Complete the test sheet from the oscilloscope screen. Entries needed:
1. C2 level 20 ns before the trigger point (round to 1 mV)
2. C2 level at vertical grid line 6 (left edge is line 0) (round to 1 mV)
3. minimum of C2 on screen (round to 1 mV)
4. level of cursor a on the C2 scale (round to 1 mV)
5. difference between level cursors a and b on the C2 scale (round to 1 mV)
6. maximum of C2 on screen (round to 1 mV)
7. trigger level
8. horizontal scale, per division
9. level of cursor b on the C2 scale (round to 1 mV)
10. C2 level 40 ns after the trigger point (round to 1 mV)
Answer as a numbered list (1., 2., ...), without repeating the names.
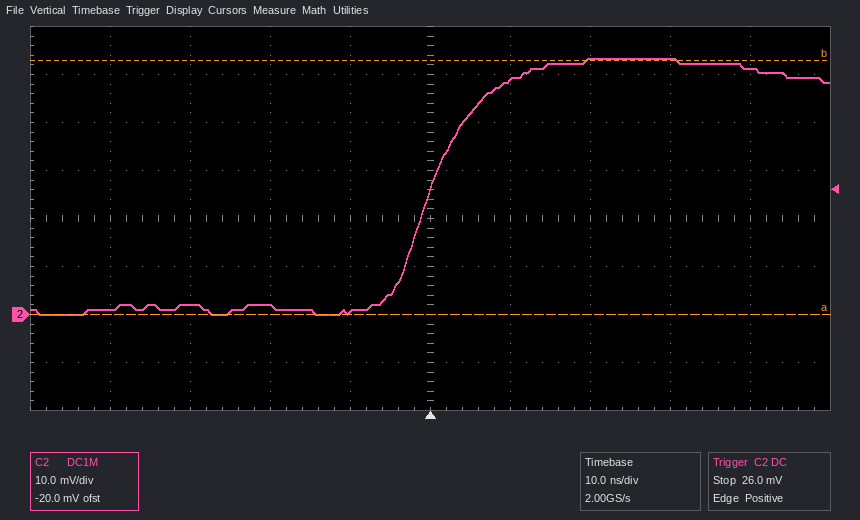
1. 2 mV
2. 49 mV
3. 0 mV
4. 0 mV
5. 53 mV
6. 53 mV
7. 26.0 mV
8. 10 ns
9. 53 mV
10. 51 mV
